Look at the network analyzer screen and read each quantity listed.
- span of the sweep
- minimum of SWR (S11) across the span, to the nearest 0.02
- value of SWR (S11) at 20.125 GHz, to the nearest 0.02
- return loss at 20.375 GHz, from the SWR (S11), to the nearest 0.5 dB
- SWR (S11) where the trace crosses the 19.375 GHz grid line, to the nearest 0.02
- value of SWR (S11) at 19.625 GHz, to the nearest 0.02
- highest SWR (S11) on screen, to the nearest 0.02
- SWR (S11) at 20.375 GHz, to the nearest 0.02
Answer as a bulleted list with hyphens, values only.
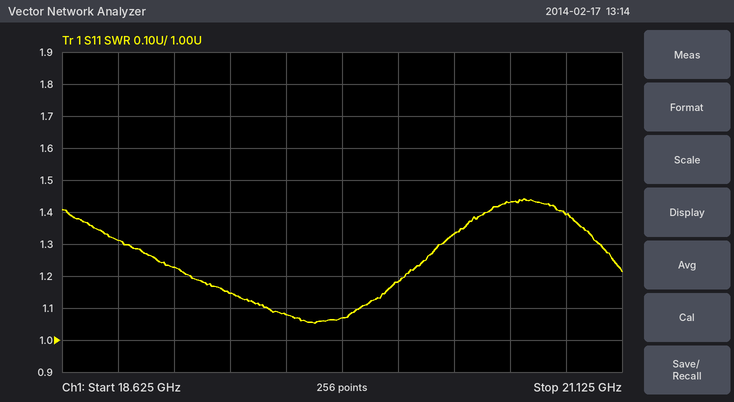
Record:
- 2.5 GHz
- 1.06
- 1.18
- 17.0 dB
- 1.14
- 1.08
- 1.44
- 1.34
